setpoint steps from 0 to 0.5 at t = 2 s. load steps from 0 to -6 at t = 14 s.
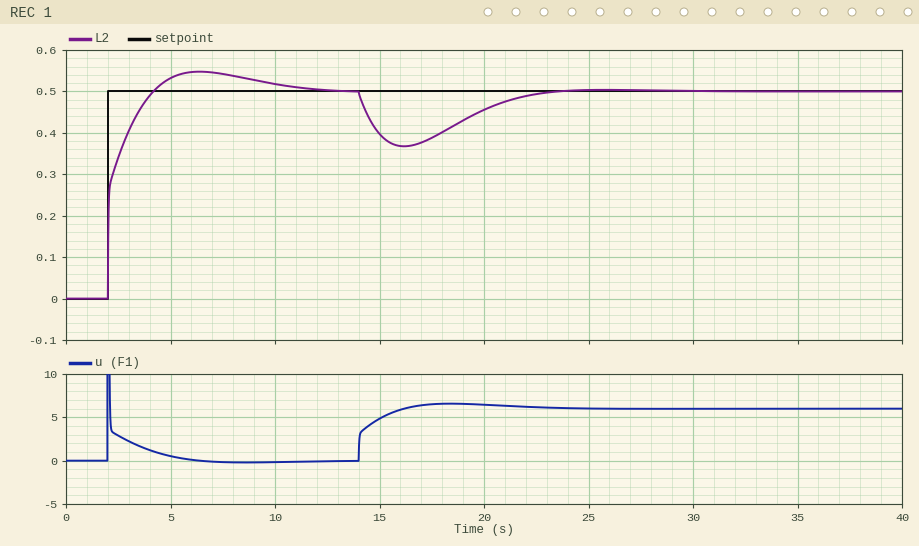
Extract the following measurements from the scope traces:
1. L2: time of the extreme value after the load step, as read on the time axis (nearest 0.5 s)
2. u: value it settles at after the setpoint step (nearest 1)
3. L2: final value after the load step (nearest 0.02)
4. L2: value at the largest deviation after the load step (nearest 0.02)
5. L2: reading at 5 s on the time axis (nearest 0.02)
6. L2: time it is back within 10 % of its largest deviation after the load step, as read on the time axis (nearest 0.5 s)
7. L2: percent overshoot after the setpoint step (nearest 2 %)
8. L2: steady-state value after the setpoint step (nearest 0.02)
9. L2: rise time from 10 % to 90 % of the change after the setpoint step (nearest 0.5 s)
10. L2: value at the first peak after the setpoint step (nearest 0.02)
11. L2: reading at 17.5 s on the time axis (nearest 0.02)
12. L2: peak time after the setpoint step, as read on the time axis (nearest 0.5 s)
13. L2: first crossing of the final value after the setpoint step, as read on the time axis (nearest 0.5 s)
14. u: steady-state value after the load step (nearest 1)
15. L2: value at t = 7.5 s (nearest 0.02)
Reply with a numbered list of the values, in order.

1. 16.0 s
2. 0
3. 0.50
4. 0.36
5. 0.54
6. 22.0 s
7. 10 %
8. 0.50
9. 1.5 s
10. 0.54
11. 0.38
12. 6.5 s
13. 4.0 s
14. 6
15. 0.54
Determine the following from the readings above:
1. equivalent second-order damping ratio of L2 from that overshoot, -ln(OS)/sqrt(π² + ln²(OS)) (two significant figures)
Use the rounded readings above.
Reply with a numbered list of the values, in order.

1. 0.59
